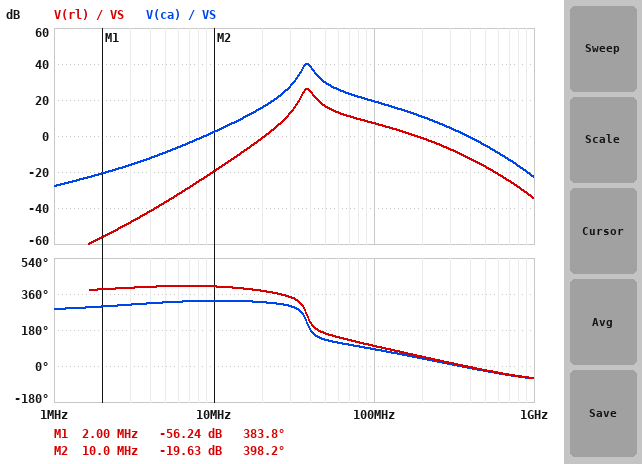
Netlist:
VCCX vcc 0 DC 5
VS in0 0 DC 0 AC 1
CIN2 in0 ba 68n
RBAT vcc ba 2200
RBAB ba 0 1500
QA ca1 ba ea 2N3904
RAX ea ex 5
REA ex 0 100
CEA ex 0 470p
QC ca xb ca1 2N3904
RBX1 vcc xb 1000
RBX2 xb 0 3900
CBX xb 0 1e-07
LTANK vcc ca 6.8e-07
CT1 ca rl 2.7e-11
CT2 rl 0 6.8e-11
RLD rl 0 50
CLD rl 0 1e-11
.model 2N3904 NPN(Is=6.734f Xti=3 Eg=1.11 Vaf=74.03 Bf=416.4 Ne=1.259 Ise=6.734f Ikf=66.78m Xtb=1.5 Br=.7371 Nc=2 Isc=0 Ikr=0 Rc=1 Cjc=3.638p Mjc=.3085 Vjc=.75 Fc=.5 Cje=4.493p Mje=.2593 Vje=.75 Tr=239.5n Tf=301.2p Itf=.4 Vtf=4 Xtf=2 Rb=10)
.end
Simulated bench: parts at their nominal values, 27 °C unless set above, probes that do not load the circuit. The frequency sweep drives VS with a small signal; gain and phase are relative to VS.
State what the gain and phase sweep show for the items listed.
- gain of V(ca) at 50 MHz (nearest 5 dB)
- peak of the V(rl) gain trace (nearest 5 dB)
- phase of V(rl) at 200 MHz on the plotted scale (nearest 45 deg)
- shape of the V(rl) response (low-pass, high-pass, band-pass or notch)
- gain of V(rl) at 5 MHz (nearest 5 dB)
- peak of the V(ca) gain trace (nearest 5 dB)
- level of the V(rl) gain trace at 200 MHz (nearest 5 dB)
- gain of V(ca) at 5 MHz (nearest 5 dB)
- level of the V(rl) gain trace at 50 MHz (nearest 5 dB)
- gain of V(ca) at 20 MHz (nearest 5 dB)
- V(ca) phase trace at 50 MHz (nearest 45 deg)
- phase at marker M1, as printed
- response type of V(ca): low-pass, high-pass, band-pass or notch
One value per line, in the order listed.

30 dB
25 dB
45 deg
band-pass
-35 dB
40 dB
0 dB
-10 dB
15 dB
15 dB
135 deg
383.8 deg
band-pass
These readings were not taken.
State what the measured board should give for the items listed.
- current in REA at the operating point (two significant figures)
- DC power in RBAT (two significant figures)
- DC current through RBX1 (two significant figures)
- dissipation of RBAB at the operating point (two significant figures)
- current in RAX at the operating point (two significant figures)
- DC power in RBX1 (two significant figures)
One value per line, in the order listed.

12 mA
4.2 mW
1.1 mA
2.6 mW
12 mA
1.2 mW
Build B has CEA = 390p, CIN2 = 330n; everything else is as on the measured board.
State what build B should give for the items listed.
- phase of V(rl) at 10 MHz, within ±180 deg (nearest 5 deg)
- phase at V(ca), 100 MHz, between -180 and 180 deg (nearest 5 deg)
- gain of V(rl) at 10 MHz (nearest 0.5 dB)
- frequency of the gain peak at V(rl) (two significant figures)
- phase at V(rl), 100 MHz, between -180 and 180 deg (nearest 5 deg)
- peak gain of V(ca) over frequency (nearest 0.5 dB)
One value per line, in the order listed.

35 deg
90 deg
-21.0 dB
38 MHz
105 deg
39.0 dB
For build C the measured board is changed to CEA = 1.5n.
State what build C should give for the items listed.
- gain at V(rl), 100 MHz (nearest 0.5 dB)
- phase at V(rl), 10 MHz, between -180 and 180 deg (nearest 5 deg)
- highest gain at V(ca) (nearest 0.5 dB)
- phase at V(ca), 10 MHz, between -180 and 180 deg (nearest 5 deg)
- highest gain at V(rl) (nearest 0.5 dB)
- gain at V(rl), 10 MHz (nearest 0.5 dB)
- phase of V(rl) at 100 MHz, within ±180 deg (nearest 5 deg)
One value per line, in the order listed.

7.5 dB
30 deg
43.5 dB
-45 deg
29.5 dB
-11.5 dB
85 deg
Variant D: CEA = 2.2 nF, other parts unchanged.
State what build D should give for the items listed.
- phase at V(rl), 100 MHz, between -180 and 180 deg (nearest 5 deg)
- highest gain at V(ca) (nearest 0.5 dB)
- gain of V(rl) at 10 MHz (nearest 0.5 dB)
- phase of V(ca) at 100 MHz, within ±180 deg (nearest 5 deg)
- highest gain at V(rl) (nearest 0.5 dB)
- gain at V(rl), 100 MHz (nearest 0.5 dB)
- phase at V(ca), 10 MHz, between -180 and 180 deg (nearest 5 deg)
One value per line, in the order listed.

80 deg
44.0 dB
-9.5 dB
65 deg
30.0 dB
7.5 dB
-50 deg
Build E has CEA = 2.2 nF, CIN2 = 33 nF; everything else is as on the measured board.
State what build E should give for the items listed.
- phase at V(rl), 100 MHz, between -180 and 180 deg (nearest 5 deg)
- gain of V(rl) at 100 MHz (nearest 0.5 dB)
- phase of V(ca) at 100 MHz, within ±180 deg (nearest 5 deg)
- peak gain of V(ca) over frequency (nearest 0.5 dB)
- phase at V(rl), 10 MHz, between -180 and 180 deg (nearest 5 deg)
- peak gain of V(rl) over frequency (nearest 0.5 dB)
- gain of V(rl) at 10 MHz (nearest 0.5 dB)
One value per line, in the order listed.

80 deg
7.5 dB
65 deg
44.0 dB
20 deg
30.0 dB
-9.5 dB
